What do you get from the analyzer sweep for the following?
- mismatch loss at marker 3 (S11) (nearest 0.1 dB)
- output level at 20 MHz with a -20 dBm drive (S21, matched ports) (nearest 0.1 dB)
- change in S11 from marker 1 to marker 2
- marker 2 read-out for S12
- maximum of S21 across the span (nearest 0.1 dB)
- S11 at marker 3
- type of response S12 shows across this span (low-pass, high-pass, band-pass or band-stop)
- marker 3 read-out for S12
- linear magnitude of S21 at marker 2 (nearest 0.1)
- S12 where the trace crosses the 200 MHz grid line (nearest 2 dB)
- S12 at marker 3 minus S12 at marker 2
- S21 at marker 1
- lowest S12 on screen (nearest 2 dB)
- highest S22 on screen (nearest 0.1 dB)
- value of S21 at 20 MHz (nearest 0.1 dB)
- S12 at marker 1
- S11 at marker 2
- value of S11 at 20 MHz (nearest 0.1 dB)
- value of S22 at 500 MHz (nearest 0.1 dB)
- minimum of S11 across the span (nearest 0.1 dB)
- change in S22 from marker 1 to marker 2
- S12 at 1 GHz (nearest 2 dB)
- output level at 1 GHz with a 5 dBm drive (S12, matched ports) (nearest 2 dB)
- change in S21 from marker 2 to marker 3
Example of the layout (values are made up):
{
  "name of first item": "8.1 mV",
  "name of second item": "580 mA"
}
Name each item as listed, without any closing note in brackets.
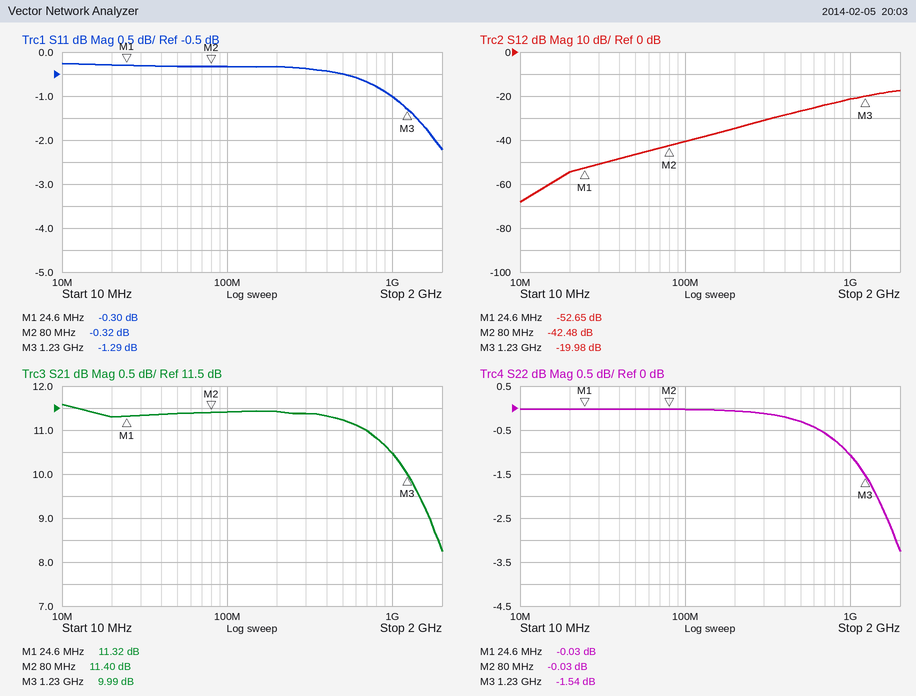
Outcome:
{
  "mismatch loss at marker 3 (S11)": "5.9 dB",
  "output level at 20 MHz with a -20 dBm drive (S21, matched ports)": "-8.7 dBm",
  "change in S11 from marker 1 to marker 2": "-0.02 dB",
  "marker 2 read-out for S12": "-42.48 dB",
  "maximum of S21 across the span": "11.6 dB",
  "S11 at marker 3": "-1.29 dB",
  "type of response S12 shows across this span": "high-pass",
  "marker 3 read-out for S12": "-19.98 dB",
  "linear magnitude of S21 at marker 2": "3.7",
  "S12 where the trace crosses the 200 MHz grid line": "-34 dB",
  "S12 at marker 3 minus S12 at marker 2": "22.50 dB",
  "S21 at marker 1": "11.32 dB",
  "lowest S12 on screen": "-68 dB",
  "highest S22 on screen": "0.0 dB",
  "value of S21 at 20 MHz": "11.3 dB",
  "S12 at marker 1": "-52.65 dB",
  "S11 at marker 2": "-0.32 dB",
  "value of S11 at 20 MHz": "-0.3 dB",
  "value of S22 at 500 MHz": "-0.3 dB",
  "minimum of S11 across the span": "-2.2 dB",
  "change in S22 from marker 1 to marker 2": "0.00 dB",
  "S12 at 1 GHz": "-22 dB",
  "output level at 1 GHz with a 5 dBm drive (S12, matched ports)": "-16 dBm",
  "change in S21 from marker 2 to marker 3": "-1.41 dB"
}
